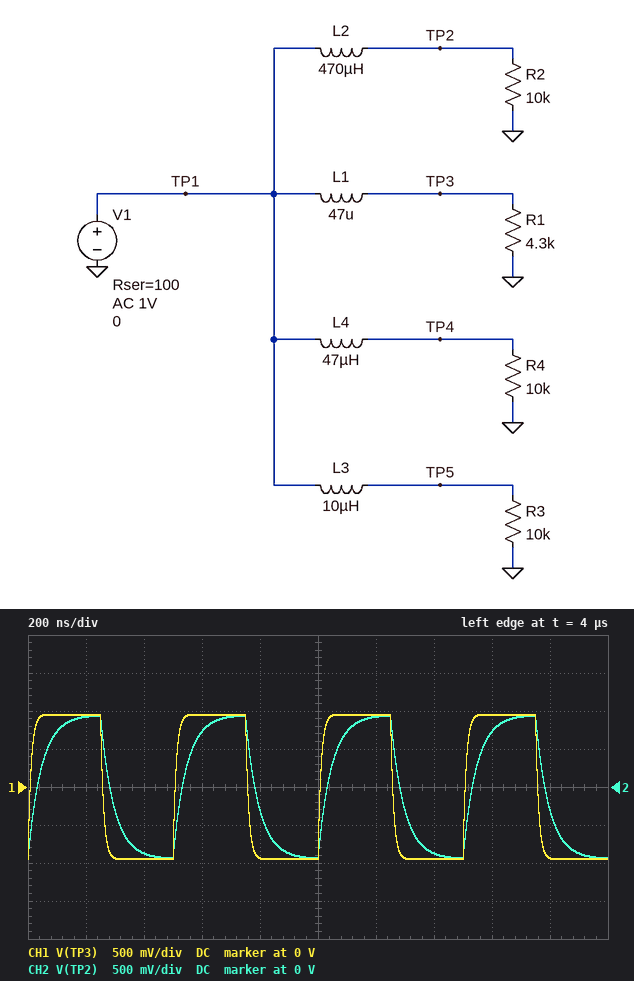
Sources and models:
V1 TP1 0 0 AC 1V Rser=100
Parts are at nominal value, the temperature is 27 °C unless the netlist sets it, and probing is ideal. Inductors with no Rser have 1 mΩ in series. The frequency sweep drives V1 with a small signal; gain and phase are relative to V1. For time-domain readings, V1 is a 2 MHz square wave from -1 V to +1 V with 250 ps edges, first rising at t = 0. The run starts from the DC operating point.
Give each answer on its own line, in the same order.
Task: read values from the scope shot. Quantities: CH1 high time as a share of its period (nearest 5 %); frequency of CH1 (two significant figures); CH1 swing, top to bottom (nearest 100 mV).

50 %
2.0 MHz
1.9 V
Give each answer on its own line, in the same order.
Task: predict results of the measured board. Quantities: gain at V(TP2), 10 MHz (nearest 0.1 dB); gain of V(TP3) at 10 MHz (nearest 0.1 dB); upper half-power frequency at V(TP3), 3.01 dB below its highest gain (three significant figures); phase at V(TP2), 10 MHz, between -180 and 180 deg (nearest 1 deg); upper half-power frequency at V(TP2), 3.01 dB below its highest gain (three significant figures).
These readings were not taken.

-10.2 dB
-2.0 dB
15.2 MHz
-70 deg
3.43 MHz
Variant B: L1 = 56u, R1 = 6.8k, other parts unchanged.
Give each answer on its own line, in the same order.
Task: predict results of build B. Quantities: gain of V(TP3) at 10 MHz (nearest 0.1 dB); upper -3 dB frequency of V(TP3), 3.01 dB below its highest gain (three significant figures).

-1.3 dB
20.1 MHz
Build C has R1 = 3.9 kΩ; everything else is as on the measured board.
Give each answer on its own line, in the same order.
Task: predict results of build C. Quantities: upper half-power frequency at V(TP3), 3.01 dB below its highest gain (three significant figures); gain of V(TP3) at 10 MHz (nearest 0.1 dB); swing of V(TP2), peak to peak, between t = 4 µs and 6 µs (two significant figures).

13.8 MHz
-2.3 dB
1.9 V
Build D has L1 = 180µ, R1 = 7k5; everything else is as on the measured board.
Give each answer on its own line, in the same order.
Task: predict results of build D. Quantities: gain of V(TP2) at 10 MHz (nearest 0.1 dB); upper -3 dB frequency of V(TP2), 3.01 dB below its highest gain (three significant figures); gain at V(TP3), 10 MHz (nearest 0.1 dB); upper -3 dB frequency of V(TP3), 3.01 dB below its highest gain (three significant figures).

-10.1 dB
3.44 MHz
-5.4 dB
6.83 MHz
